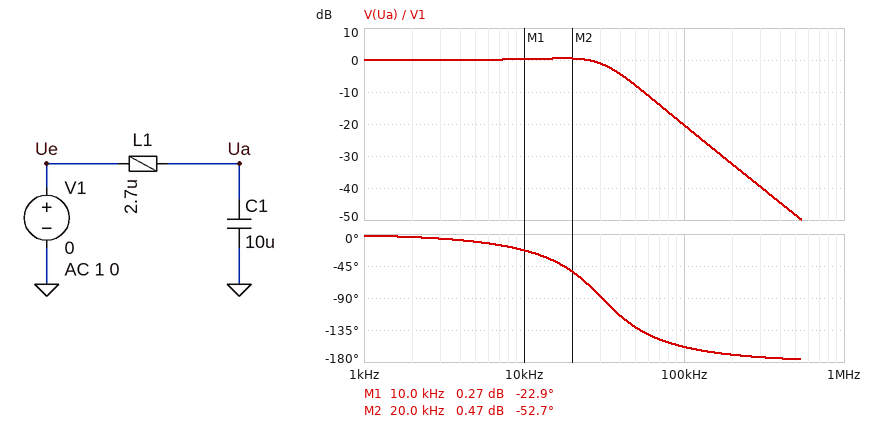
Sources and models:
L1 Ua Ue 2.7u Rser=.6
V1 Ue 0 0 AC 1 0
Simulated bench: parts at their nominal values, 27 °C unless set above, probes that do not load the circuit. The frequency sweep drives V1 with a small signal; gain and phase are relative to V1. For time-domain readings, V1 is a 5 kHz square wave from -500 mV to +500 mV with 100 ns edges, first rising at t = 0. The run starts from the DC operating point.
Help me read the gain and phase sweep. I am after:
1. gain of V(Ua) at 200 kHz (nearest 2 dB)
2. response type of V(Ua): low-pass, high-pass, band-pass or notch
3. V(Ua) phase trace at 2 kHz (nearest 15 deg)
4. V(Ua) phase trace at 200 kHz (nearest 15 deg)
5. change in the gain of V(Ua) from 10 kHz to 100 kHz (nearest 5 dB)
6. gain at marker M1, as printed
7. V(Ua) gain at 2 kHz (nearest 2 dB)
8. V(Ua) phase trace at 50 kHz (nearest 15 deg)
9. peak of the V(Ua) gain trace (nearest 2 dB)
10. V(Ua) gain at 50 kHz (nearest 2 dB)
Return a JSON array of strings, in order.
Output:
["-32 dB", "low-pass", "0 deg", "-165 deg", "-20 dB", "0.27 dB", "0 dB", "-135 deg", "0 dB", "-8 dB"]
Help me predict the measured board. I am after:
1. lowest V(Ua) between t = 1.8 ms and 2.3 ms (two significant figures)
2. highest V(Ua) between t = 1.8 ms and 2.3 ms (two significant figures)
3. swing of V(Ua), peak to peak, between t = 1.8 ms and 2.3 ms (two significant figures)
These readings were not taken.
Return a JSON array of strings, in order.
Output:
["-610 mV", "610 mV", "1.2 V"]
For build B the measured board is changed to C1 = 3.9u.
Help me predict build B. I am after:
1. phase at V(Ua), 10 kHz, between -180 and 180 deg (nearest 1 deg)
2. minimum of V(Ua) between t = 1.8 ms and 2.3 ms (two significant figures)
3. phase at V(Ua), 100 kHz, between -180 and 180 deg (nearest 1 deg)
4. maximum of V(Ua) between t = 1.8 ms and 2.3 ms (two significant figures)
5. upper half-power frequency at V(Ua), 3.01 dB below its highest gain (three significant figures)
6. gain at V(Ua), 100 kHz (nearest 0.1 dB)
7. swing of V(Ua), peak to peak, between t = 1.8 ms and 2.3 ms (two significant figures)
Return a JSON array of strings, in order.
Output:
["-9 deg", "-800 mV", "-155 deg", "800 mV", "58.3 kHz", "-10.8 dB", "1.6 V"]
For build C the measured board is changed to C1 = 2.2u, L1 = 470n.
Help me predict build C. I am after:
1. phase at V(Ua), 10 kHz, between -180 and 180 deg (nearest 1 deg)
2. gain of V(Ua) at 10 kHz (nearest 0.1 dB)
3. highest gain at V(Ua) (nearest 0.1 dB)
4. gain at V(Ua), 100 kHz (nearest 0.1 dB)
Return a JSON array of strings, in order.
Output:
["-5 deg", "0 dB", "0.1 dB", "-0.2 dB"]
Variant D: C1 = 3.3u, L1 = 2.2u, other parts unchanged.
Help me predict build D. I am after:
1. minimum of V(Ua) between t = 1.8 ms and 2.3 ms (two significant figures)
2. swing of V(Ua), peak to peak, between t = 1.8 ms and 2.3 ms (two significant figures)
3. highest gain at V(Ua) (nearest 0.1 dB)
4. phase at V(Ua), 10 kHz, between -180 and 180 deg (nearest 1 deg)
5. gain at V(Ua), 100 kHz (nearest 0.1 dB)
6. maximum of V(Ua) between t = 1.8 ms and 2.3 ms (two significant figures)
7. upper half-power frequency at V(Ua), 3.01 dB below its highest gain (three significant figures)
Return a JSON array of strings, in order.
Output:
["-790 mV", "1.6 V", "3.3 dB", "-7 deg", "-7.0 dB", "790 mV", "70.2 kHz"]
